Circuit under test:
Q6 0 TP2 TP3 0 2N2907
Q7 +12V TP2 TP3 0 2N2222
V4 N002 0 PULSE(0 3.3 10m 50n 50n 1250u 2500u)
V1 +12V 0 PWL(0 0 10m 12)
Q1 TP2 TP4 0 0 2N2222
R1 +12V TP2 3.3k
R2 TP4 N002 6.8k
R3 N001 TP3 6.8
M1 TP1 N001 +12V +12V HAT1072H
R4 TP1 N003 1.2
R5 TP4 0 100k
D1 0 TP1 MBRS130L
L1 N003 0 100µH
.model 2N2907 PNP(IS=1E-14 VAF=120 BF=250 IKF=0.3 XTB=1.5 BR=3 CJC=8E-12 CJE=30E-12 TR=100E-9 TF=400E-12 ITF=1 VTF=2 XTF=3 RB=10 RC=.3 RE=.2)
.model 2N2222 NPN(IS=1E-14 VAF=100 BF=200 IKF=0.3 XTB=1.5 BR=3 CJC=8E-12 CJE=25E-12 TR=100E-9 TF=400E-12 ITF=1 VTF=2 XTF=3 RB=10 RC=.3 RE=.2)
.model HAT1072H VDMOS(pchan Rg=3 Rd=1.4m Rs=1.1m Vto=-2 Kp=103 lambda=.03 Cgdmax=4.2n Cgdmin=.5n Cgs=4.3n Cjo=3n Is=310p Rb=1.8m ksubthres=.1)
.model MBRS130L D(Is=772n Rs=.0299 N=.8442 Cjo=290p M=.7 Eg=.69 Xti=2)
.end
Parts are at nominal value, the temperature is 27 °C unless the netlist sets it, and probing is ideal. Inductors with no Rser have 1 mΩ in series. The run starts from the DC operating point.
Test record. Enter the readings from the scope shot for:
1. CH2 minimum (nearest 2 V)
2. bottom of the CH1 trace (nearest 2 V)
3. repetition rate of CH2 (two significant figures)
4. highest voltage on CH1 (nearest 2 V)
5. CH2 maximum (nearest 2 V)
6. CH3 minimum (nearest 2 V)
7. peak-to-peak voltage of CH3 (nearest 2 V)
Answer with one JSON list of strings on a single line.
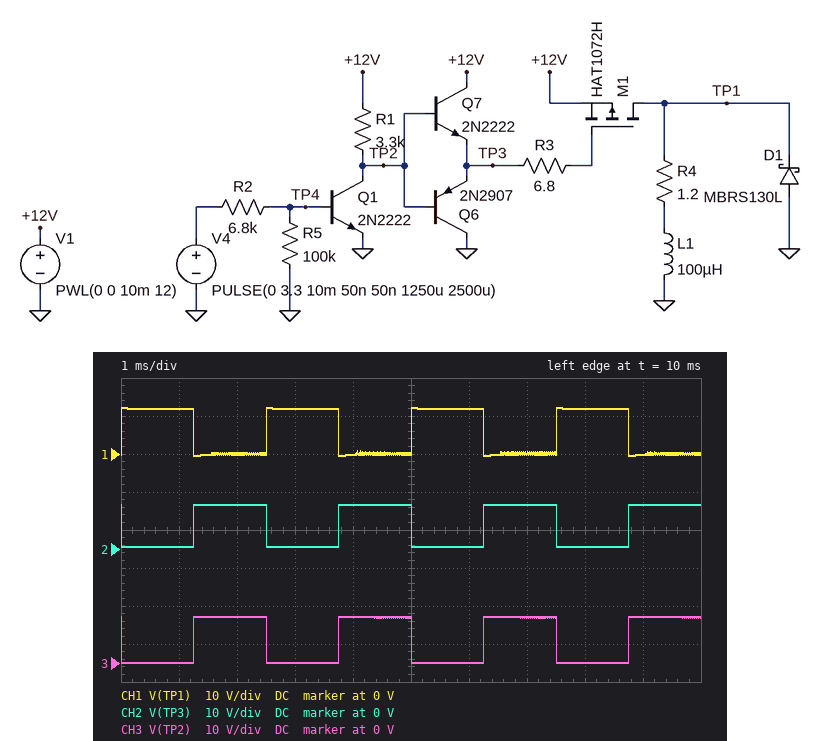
["0 V", "0 V", "400 Hz", "12 V", "12 V", "0 V", "12 V"]
